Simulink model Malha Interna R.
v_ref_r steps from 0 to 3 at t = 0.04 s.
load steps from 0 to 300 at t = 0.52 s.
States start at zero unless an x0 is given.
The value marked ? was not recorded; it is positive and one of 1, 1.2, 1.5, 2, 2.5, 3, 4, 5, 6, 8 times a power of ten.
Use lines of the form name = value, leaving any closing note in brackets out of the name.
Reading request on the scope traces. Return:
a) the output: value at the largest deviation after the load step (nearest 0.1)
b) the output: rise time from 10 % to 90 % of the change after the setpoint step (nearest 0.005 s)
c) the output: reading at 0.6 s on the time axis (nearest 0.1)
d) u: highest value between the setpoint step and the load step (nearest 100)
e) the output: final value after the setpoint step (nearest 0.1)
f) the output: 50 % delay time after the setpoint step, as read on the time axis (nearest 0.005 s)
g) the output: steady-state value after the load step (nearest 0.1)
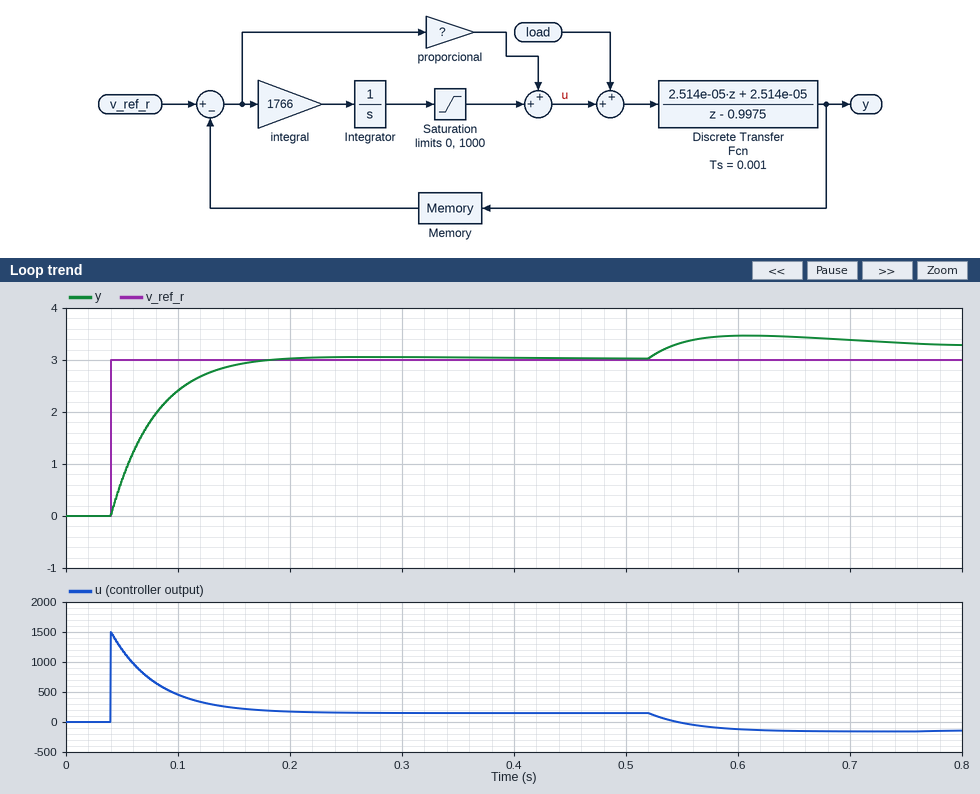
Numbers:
the output: value at the largest deviation after the load step = 3.5
the output: rise time from 10 % to 90 % of the change after the setpoint step = 0.080 s
the output: reading at 0.6 s on the time axis = 3.5
u: highest value between the setpoint step and the load step = 1500
the output: final value after the setpoint step = 3.0
the output: 50 % delay time after the setpoint step, as read on the time axis = 0.065 s
the output: steady-state value after the load step = 3.3
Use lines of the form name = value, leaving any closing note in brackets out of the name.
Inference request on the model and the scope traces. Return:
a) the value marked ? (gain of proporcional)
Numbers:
the value marked ? = 500
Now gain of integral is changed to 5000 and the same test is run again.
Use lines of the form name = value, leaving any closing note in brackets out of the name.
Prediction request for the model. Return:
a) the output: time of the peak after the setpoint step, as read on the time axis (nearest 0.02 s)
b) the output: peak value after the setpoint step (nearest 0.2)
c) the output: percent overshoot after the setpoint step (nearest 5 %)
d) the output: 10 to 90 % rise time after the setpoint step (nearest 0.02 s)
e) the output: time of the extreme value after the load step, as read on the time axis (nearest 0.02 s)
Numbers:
the output: time of the peak after the setpoint step, as read on the time axis = 0.18 s
the output: peak value after the setpoint step = 3.4
the output: percent overshoot after the setpoint step = 10 %
the output: 10 to 90 % rise time after the setpoint step = 0.06 s
the output: time of the extreme value after the load step, as read on the time axis = 0.58 s
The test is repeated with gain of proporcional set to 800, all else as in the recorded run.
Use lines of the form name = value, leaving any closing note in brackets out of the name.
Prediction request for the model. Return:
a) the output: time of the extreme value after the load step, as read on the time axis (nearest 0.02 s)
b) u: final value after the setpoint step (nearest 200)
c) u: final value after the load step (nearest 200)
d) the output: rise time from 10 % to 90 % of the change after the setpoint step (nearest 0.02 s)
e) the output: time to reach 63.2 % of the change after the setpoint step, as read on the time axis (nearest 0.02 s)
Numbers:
the output: time of the extreme value after the load step, as read on the time axis = 0.60 s
u: final value after the setpoint step = 200
u: final value after the load step = -200
the output: rise time from 10 % to 90 % of the change after the setpoint step = 0.06 s
the output: time to reach 63.2 % of the change after the setpoint step, as read on the time axis = 0.06 s
